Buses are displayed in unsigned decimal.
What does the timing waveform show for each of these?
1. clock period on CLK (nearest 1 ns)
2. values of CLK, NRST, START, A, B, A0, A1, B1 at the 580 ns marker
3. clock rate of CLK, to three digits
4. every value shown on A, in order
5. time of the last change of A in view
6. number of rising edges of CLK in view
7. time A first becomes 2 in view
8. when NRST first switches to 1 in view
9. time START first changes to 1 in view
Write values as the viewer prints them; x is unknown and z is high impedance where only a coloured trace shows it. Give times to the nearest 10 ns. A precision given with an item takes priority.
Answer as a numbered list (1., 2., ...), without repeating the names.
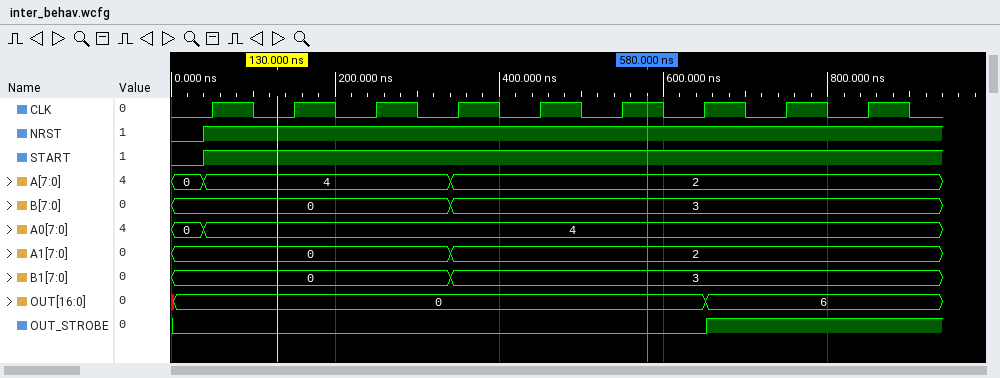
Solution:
1. 100 ns
2. CLK=1, NRST=1, START=1, A=2, B=3, A0=4, A1=2, B1=3
3. 10.0 MHz
4. 0, 4, 2
5. 340 ns
6. 9
7. 340 ns
8. 40 ns
9. 40 ns
